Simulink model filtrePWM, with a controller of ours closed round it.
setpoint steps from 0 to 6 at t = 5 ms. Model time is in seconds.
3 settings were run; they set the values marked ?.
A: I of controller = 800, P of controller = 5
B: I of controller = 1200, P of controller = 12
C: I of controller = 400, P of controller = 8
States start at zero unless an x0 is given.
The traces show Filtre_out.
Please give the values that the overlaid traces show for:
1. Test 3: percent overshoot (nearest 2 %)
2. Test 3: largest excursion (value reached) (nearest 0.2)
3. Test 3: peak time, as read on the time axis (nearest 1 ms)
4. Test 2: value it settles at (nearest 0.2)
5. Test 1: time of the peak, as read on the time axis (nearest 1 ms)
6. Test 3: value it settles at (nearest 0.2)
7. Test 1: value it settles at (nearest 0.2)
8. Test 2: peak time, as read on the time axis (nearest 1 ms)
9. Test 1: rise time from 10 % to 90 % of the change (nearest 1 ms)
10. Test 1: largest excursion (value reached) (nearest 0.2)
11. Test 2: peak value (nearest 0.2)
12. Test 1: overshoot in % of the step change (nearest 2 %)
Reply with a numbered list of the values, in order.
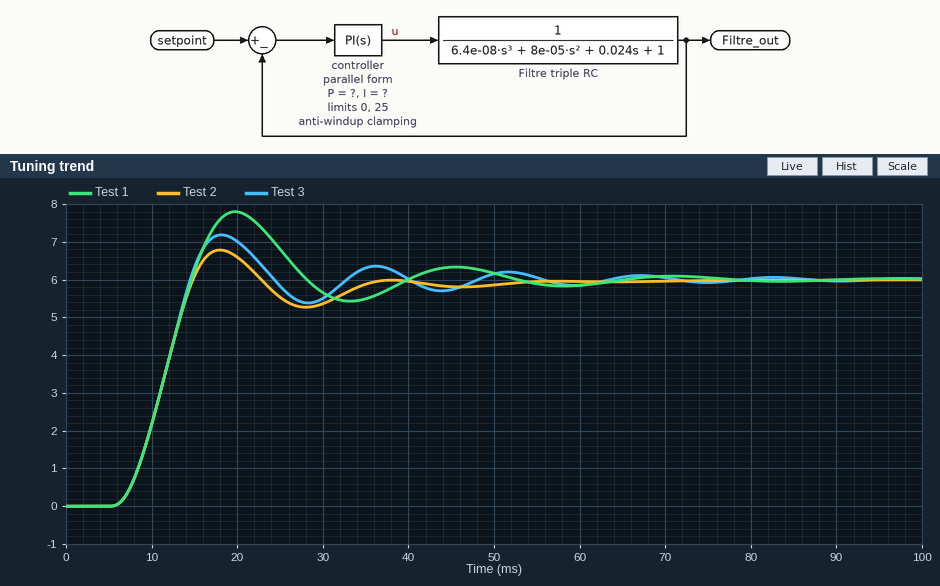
1. 20 %
2. 7.2
3. 18 ms
4. 6.0
5. 20 ms
6. 6.0
7. 6.0
8. 18 ms
9. 6 ms
10. 7.8
11. 6.8
12. 30 %
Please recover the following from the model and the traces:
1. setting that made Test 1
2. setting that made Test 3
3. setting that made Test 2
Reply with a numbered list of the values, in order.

1. A
2. B
3. C
